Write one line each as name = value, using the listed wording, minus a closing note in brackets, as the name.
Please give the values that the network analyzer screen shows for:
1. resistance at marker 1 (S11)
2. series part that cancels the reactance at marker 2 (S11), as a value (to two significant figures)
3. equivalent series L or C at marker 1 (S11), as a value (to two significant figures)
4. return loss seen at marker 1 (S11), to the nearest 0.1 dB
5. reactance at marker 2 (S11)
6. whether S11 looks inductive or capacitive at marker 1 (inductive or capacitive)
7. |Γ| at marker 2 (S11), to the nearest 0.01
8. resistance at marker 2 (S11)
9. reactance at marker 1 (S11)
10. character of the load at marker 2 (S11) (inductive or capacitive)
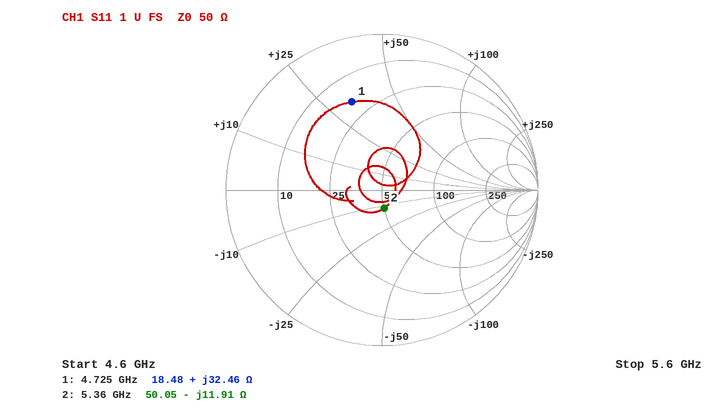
resistance at marker 1 = 18.48 Ω
series part that cancels the reactance at marker 2 (S11), as a value = 350 pH
equivalent series L or C at marker 1 (S11), as a value = 1.1 nH
return loss seen at marker 1 (S11), to the nearest 0.1 dB = 4.5 dB
reactance at marker 2 = -11.91 Ω
whether S11 looks inductive or capacitive at marker 1 = inductive
|Γ| at marker 2 (S11), to the nearest 0.01 = 0.12
resistance at marker 2 = 50.05 Ω
reactance at marker 1 = +32.46 Ω
character of the load at marker 2 (S11) = capacitive
